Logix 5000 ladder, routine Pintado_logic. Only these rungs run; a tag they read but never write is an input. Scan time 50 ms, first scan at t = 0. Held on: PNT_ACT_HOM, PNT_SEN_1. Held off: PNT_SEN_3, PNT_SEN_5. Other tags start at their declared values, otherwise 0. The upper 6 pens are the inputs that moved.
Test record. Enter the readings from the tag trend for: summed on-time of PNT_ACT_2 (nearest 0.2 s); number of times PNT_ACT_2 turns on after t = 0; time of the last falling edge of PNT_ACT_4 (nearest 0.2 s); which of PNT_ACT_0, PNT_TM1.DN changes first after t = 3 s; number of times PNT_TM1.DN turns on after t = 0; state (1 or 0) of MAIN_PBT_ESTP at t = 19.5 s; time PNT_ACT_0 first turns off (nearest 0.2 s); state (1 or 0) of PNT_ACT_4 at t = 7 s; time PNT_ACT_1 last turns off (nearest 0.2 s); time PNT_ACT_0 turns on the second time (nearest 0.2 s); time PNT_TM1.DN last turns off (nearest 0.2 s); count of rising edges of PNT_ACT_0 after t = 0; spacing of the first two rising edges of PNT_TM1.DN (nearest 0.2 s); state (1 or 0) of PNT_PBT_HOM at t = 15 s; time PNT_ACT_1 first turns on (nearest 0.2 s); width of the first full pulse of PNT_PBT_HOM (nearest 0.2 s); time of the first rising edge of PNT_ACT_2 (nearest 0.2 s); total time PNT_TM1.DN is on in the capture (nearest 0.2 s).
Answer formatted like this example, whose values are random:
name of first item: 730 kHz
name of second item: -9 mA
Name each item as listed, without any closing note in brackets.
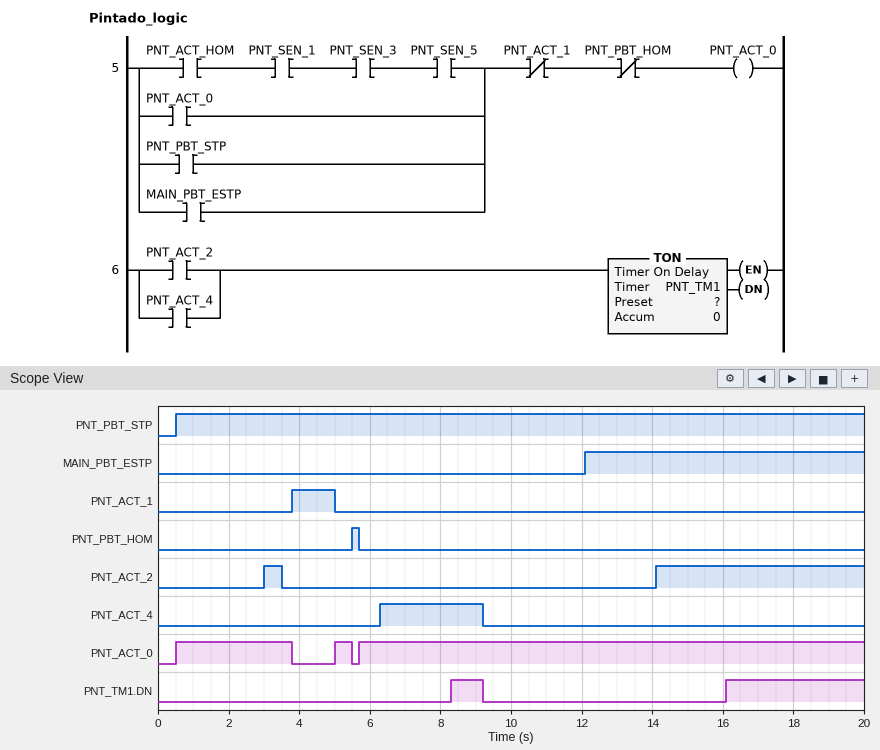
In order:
summed on-time of PNT_ACT_2: 6.4 s
number of times PNT_ACT_2 turns on after t = 0: 2
time of the last falling edge of PNT_ACT_4: 9.2 s
which of PNT_ACT_0, PNT_TM1.DN changes first after t = 3 s: PNT_ACT_0
number of times PNT_TM1.DN turns on after t = 0: 2
state (1 or 0) of MAIN_PBT_ESTP at t = 19.5 s: 1
time PNT_ACT_0 first turns off: 3.8 s
state (1 or 0) of PNT_ACT_4 at t = 7 s: 1
time PNT_ACT_1 last turns off: 5.0 s
time PNT_ACT_0 turns on the second time: 5.0 s
time PNT_TM1.DN last turns off: 9.2 s
count of rising edges of PNT_ACT_0 after t = 0: 3
spacing of the first two rising edges of PNT_TM1.DN: 7.8 s
state (1 or 0) of PNT_PBT_HOM at t = 15 s: 0
time PNT_ACT_1 first turns on: 3.8 s
width of the first full pulse of PNT_PBT_HOM: 0.2 s
time of the first rising edge of PNT_ACT_2: 3.0 s
total time PNT_TM1.DN is on in the capture: 4.8 s
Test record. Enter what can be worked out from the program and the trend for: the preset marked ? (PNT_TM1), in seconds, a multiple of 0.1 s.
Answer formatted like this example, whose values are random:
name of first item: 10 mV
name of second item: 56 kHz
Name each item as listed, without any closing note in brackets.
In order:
the preset marked ? (PNT_TM1), in seconds, a multiple of 0.1 s: 2.0 s
